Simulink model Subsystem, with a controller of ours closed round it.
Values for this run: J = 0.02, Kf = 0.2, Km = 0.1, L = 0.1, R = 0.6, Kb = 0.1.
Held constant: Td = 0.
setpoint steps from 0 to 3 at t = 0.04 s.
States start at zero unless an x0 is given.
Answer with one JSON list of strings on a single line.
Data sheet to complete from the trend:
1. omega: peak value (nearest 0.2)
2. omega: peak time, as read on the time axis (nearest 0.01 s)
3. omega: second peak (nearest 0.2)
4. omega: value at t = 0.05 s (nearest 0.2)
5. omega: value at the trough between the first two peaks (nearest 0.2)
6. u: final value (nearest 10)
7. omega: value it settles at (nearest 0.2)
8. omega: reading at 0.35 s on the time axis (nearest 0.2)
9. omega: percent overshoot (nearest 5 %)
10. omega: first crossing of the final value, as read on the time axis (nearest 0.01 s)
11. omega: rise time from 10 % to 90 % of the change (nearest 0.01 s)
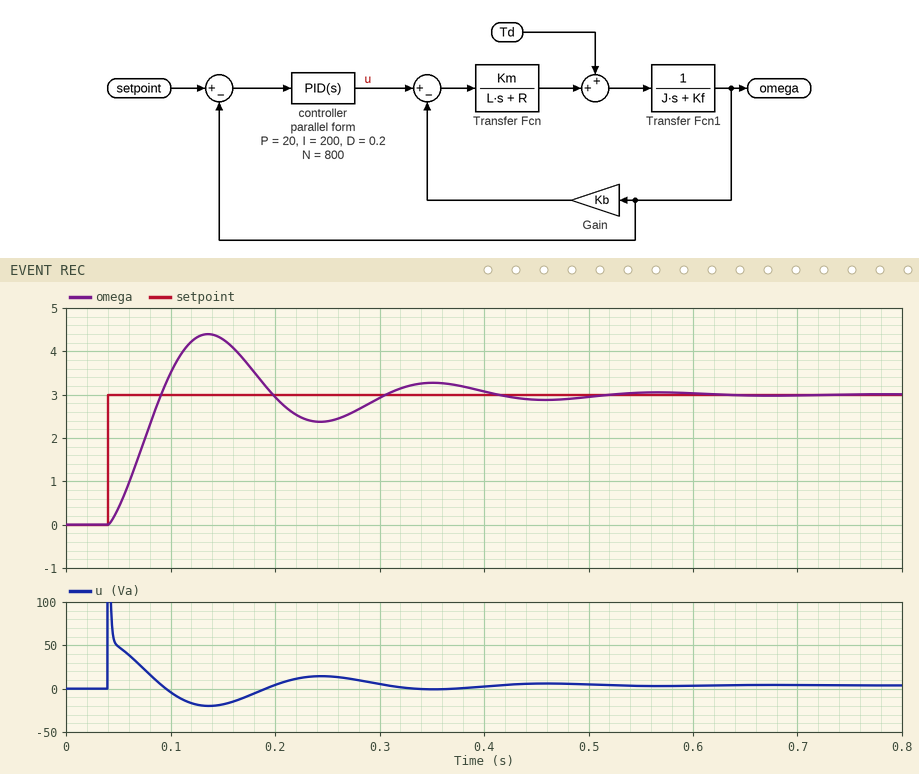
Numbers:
["4.4", "0.14 s", "3.2", "0.4", "2.4", "0", "3.0", "3.2", "45 %", "0.09 s", "0.04 s"]
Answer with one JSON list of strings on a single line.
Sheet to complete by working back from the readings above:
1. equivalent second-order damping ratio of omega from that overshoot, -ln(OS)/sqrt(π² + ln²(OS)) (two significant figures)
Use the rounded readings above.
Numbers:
["0.25"]
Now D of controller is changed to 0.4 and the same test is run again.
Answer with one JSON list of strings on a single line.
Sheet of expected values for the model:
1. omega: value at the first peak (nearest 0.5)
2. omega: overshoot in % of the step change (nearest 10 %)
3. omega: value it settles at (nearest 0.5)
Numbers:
["4.0", "30 %", "3.0"]
